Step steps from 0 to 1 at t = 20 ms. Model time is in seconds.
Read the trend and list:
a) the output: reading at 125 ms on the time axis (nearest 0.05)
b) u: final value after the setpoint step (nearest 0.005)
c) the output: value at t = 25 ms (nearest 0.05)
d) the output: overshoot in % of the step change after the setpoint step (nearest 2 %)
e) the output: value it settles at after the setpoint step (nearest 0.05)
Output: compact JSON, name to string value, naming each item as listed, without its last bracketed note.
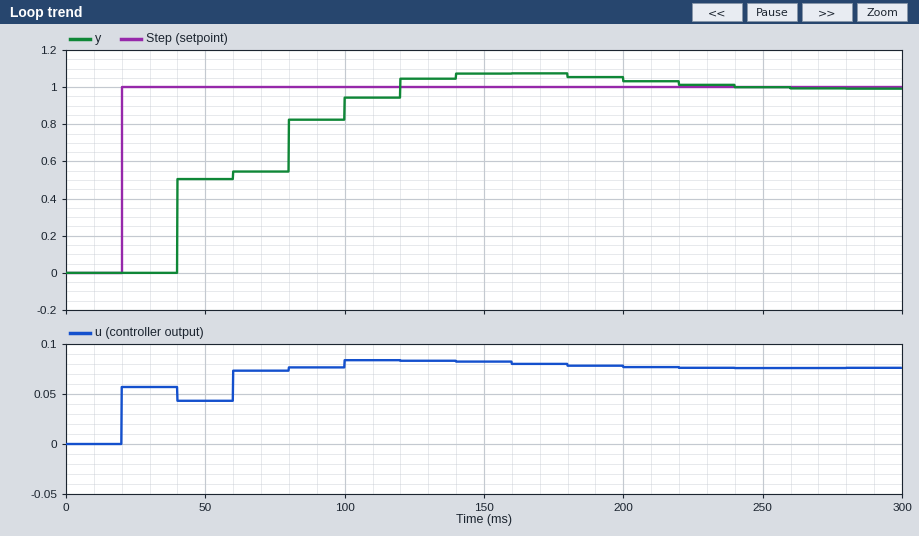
{"the output: reading at 125 ms on the time axis": "1.05", "u: final value after the setpoint step": "0.075", "the output: value at t = 25 ms": "0.00", "the output: overshoot in % of the step change after the setpoint step": "8 %", "the output: value it settles at after the setpoint step": "1.00"}
